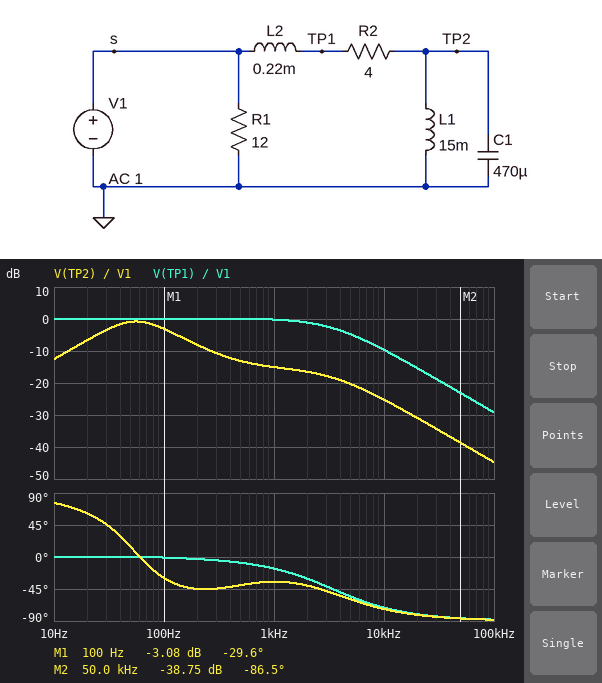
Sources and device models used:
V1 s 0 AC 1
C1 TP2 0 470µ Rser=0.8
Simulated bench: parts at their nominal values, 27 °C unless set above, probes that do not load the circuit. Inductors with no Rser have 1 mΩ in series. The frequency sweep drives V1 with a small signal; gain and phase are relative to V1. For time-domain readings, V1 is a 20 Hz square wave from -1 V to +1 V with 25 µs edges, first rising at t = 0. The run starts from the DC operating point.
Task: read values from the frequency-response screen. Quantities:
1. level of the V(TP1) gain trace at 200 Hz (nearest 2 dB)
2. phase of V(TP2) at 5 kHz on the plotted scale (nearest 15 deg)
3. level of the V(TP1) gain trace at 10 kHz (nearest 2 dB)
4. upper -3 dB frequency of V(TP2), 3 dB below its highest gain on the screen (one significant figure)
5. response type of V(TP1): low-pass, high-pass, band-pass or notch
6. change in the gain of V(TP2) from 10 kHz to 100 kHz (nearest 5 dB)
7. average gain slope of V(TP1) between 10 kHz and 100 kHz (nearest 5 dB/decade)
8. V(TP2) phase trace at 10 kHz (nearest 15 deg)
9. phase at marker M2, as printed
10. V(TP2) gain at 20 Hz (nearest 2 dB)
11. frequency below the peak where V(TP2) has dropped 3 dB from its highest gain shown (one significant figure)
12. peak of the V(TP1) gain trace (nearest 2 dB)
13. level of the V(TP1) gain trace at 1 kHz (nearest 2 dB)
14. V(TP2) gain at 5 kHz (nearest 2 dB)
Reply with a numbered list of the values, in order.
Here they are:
1. 0 dB
2. -60 deg
3. -10 dB
4. 100 Hz
5. low-pass
6. -20 dB
7. -20 dB/decade
8. -75 deg
9. -86.5 deg
10. -6 dB
11. 30 Hz
12. 0 dB
13. 0 dB
14. -20 dB
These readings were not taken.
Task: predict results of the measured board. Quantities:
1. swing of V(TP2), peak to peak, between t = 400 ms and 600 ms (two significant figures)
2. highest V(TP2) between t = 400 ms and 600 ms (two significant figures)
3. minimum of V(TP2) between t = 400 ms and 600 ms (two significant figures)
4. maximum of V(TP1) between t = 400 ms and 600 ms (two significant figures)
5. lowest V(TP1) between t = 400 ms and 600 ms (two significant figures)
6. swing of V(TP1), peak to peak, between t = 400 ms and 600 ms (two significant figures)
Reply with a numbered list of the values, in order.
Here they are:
1. 2.4 V
2. 1.2 V
3. -1.2 V
4. 1.0 V
5. -1.0 V
6. 2.1 V
